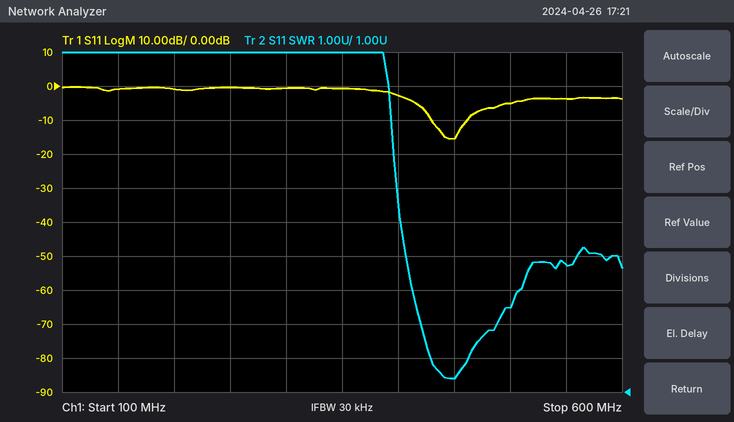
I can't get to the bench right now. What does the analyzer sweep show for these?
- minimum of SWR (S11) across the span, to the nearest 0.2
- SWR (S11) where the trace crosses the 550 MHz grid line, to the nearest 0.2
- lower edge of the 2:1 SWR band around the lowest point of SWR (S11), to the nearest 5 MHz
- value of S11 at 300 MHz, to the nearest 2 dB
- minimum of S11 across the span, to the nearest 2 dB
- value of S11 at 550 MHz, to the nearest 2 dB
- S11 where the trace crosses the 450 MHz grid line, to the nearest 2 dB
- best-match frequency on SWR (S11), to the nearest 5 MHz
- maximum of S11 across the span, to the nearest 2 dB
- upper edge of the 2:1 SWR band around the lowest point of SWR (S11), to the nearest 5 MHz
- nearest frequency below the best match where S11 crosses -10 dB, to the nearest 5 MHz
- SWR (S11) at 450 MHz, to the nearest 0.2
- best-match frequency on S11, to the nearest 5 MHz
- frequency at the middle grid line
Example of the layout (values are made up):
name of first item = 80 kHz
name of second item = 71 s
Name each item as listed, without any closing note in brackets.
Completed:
minimum of SWR (S11) across the span, to the nearest 0.2 = 1.4
SWR (S11) where the trace crosses the 550 MHz grid line, to the nearest 0.2 = 4.8
lower edge of the 2:1 SWR band around the lowest point of SWR (S11), to the nearest 5 MHz = 430 MHz
value of S11 at 300 MHz, to the nearest 2 dB = 0 dB
minimum of S11 across the span, to the nearest 2 dB = -16 dB
value of S11 at 550 MHz, to the nearest 2 dB = -4 dB
S11 where the trace crosses the 450 MHz grid line, to the nearest 2 dB = -16 dB
best-match frequency on SWR (S11), to the nearest 5 MHz = 445 MHz
maximum of S11 across the span, to the nearest 2 dB = 0 dB
upper edge of the 2:1 SWR band around the lowest point of SWR (S11), to the nearest 5 MHz = 465 MHz
nearest frequency below the best match where S11 crosses -10 dB, to the nearest 5 MHz = 430 MHz
SWR (S11) at 450 MHz, to the nearest 0.2 = 1.4
best-match frequency on S11, to the nearest 5 MHz = 445 MHz
frequency at the middle grid line = 350 MHz
